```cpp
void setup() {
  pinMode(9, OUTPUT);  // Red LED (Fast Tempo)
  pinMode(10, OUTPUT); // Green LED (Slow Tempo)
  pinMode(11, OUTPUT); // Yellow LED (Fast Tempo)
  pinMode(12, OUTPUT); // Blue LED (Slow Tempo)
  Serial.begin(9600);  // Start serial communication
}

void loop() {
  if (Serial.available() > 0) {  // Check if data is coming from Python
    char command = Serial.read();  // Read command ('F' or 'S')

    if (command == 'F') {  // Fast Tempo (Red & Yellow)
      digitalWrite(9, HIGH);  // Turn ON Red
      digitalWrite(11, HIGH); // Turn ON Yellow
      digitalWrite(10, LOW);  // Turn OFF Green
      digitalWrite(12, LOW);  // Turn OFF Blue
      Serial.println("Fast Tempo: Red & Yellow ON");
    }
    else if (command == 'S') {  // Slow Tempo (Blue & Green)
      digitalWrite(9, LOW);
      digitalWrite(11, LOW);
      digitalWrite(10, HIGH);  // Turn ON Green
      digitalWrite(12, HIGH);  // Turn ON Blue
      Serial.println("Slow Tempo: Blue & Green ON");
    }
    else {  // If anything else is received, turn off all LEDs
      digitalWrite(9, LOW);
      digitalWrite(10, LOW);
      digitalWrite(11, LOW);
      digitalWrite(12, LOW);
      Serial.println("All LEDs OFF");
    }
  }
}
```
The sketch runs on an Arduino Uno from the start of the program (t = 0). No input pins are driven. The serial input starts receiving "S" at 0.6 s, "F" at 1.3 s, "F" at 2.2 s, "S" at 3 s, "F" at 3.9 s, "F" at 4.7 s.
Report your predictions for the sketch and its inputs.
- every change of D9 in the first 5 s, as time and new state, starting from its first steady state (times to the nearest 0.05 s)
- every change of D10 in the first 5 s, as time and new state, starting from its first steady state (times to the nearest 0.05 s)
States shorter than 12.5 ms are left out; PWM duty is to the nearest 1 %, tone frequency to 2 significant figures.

0 s low; 1.3 s high; 3 s low; 3.9 s high
0 s low; 0.6 s high; 1.3 s low; 3 s high; 3.9 s low
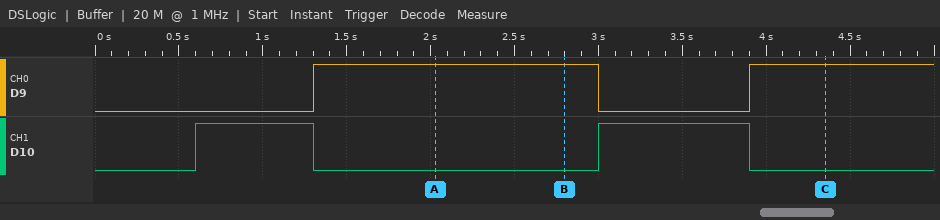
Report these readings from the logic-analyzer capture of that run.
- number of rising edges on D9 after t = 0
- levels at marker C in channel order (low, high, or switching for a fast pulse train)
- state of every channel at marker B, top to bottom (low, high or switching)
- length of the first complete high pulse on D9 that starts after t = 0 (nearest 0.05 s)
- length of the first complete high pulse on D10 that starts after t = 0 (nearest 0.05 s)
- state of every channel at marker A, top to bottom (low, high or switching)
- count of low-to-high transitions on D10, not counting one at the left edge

2
D9 high, D10 low
D9 high, D10 low
1.70 s
0.70 s
D9 high, D10 low
2
